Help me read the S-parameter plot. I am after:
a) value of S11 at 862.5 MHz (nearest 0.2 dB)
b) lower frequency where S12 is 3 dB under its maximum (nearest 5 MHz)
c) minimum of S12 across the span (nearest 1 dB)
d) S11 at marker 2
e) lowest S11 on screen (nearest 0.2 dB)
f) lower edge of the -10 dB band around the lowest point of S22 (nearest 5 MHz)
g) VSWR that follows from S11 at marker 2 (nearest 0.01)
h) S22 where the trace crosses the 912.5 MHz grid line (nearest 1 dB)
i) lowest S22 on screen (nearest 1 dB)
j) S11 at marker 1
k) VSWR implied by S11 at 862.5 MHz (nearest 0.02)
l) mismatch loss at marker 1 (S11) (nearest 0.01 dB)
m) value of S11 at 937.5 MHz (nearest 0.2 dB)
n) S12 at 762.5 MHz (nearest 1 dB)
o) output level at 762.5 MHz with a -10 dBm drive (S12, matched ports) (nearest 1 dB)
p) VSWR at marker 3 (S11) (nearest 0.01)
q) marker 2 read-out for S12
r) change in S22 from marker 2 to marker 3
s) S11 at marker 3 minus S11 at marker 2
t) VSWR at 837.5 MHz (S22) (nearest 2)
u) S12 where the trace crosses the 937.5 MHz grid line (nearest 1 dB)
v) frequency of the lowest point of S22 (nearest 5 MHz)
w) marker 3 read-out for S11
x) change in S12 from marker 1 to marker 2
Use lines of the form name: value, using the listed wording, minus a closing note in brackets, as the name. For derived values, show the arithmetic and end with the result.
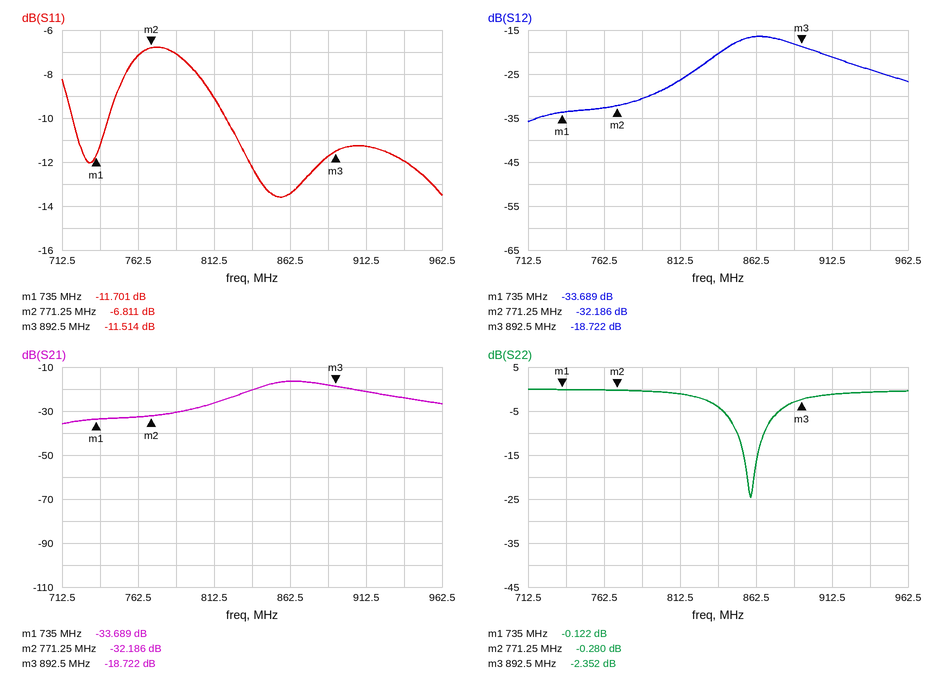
value of S11 at 862.5 MHz: -13.4 dB
lower frequency where S12 is 3 dB under its maximum: 840 MHz
minimum of S12 across the span: -36 dB
S11 at marker 2: -6.811 dB
lowest S11 on screen: -13.6 dB
lower edge of the -10 dB band around the lowest point of S22: 850 MHz
VSWR that follows from S11 at marker 2: (1 + 0.4565)/(1 − 0.4565) ≈ 2.68
S22 where the trace crosses the 912.5 MHz grid line: -1 dB
lowest S22 on screen: -25 dB
S11 at marker 1: -11.701 dB
VSWR implied by S11 at 862.5 MHz: |Γ| = 10^(-13.4/20) = 0.2138; VSWR = (1 + 0.2138)/(1 − 0.2138) ≈ 1.54
mismatch loss at marker 1 (S11): −10 log10(1 − 10^(-11.701/10)) ≈ 0.30 dB
value of S11 at 937.5 MHz: -12.0 dB
S12 at 762.5 MHz: -33 dB
output level at 762.5 MHz with a -10 dBm drive (S12, matched ports): -10 dBm + (-33 dB) = -43 dBm
VSWR at marker 3 (S11): (1 + 0.2656)/(1 − 0.2656) ≈ 1.72
marker 2 read-out for S12: -32.186 dB
change in S22 from marker 2 to marker 3: -2.352 − (-0.28) = -2.072 dB
S11 at marker 3 minus S11 at marker 2: -11.514 − (-6.811) = -4.703 dB
VSWR at 837.5 MHz (S22): |Γ| = 10^(-4/20) = 0.6310; VSWR = (1 + 0.6310)/(1 − 0.6310) ≈ 4
S12 where the trace crosses the 937.5 MHz grid line: -24 dB
frequency of the lowest point of S22: 860 MHz
marker 3 read-out for S11: -11.514 dB
change in S12 from marker 1 to marker 2: -32.186 − (-33.689) = 1.503 dB
